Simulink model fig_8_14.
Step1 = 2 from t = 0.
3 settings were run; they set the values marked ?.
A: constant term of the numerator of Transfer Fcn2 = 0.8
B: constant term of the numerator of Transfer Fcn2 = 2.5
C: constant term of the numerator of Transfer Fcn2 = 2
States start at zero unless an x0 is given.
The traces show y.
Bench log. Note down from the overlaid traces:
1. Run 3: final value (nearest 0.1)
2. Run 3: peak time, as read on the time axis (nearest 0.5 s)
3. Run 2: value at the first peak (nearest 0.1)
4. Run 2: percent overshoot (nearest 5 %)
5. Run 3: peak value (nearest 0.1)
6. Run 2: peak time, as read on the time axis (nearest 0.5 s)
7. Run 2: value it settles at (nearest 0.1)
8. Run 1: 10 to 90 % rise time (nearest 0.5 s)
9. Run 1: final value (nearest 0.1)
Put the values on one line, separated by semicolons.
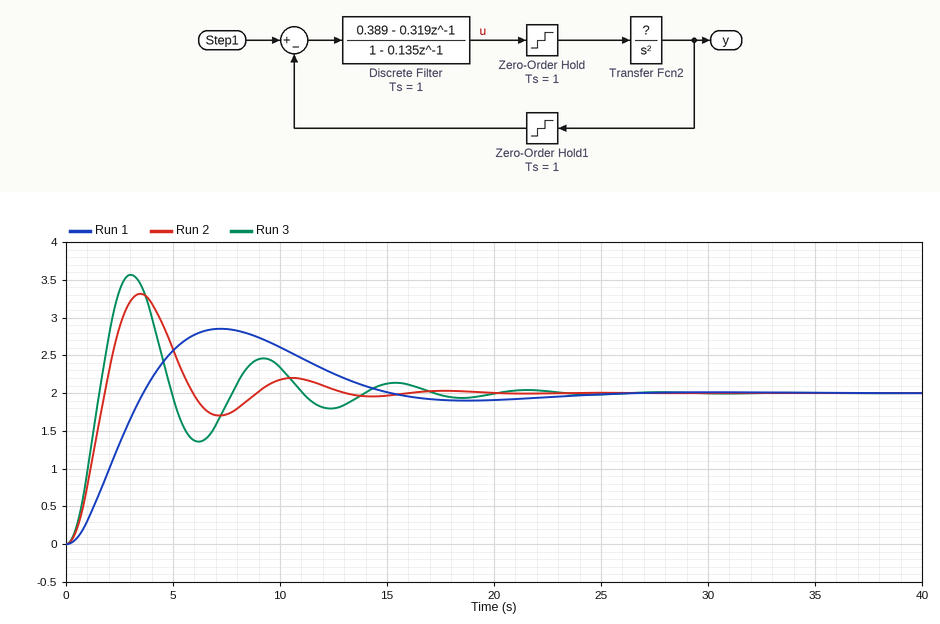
2.0; 3.0 s; 3.3; 65 %; 3.6; 3.5 s; 2.0; 2.5 s; 2.0
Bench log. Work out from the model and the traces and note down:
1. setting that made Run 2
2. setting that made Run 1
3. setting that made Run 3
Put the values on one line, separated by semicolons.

C; A; B
